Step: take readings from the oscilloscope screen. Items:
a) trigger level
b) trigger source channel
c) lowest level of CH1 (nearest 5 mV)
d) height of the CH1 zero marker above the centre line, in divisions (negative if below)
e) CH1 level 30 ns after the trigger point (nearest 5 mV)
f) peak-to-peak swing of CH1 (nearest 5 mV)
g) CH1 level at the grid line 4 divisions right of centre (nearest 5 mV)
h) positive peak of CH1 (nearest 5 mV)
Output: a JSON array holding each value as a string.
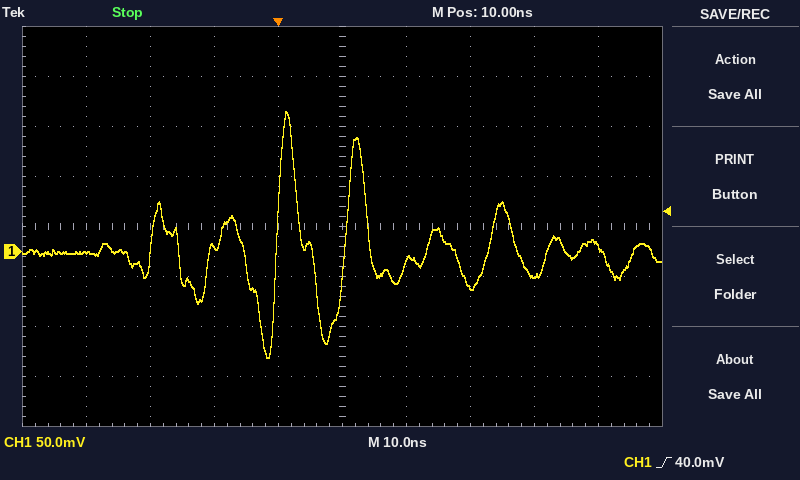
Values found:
["40.0 mV", "CH1", "-105 mV", "-0.5 div", "-35 mV", "245 mV", "5 mV", "140 mV"]
